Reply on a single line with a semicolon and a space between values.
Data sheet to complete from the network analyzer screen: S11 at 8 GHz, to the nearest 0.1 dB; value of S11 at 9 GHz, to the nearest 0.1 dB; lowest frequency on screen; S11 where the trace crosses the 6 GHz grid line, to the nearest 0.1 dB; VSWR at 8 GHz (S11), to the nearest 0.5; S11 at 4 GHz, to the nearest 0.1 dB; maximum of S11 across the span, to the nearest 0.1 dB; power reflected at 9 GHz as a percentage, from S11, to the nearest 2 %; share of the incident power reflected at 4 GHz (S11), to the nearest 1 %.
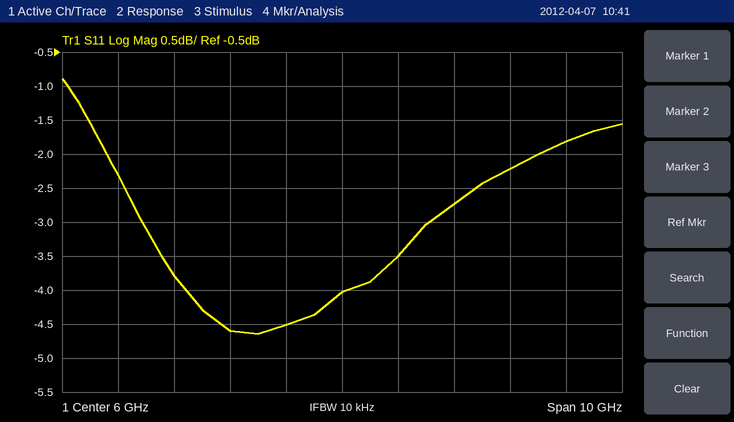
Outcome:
-2.7 dB; -2.2 dB; 1 GHz; -4.0 dB; 6.5; -4.6 dB; -0.9 dB; 60 %; 35 %
